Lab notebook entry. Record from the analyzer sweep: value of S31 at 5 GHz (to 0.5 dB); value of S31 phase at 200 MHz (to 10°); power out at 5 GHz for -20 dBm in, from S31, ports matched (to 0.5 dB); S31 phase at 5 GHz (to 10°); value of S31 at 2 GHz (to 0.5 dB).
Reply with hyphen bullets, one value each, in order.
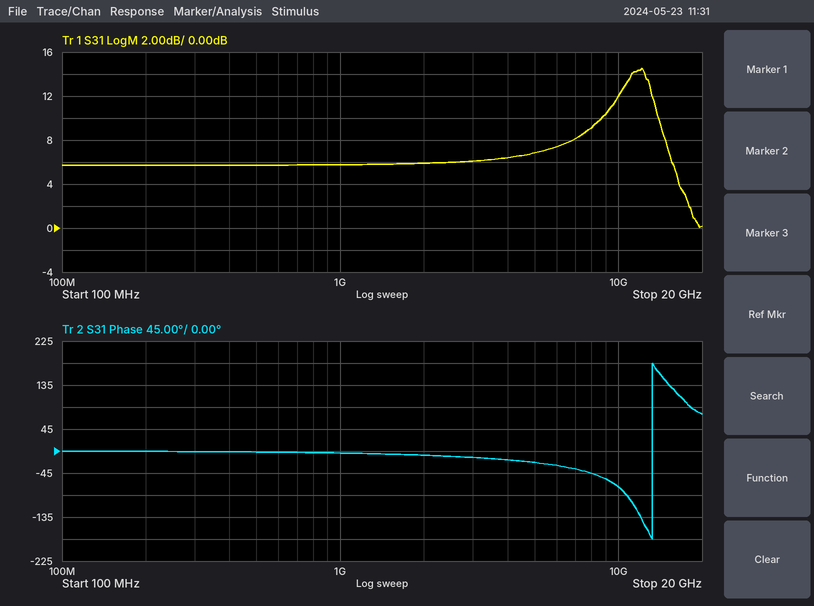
- 7.0 dB
- 0°
- -13.0 dBm
- -20°
- 6.0 dB
